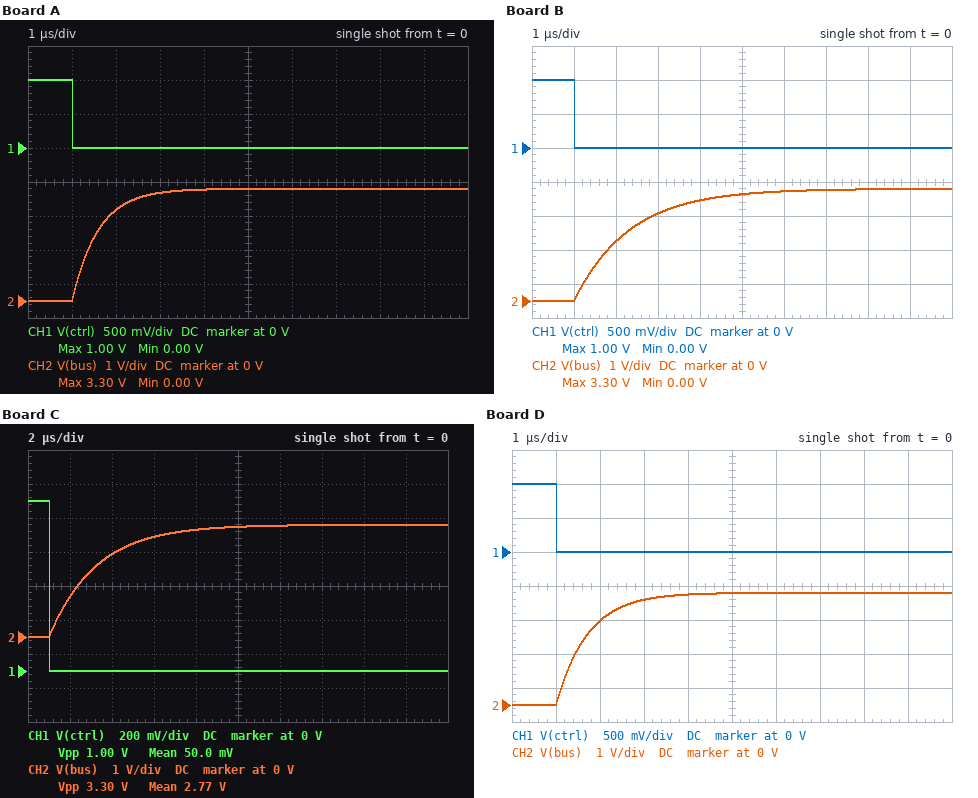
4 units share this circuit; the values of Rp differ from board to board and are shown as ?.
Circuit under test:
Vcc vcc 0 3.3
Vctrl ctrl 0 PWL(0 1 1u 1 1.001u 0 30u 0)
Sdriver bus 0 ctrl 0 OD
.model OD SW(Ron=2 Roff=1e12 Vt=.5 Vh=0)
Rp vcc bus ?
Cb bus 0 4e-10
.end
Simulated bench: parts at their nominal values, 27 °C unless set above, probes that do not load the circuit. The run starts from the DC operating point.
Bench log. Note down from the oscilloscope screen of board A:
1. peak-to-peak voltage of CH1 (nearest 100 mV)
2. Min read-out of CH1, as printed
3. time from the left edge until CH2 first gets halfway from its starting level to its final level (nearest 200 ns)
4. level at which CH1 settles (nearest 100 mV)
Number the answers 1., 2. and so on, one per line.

1. 1.0 V
2. 0.00 V
3. 1.4 µs
4. 0 V
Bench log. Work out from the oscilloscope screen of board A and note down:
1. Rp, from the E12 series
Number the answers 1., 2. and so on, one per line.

1. 1.5 kΩ
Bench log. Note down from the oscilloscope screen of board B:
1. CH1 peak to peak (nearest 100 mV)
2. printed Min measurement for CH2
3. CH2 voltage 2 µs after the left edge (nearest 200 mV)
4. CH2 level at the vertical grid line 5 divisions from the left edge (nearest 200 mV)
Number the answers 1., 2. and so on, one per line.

1. 1.0 V
2. 0.00 V
3. 1.8 V
4. 3.2 V
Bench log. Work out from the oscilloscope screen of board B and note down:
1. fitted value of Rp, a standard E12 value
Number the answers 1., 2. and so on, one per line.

1. 3.3 kΩ
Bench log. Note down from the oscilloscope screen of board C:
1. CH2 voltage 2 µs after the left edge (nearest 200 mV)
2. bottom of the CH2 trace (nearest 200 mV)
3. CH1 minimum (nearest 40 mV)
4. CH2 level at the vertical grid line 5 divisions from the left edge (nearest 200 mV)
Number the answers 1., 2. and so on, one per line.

1. 1.2 V
2. 0 V
3. 0 V
4. 3.2 V
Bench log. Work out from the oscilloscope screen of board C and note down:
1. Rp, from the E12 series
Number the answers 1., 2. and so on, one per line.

1. 5.6 kΩ
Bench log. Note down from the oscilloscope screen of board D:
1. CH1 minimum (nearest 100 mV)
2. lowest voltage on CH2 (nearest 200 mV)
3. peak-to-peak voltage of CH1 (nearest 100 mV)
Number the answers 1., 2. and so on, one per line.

1. 0 V
2. 0 V
3. 1.0 V
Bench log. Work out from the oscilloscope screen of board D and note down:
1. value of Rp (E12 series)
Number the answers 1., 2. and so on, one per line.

1. 1.8 kΩ
